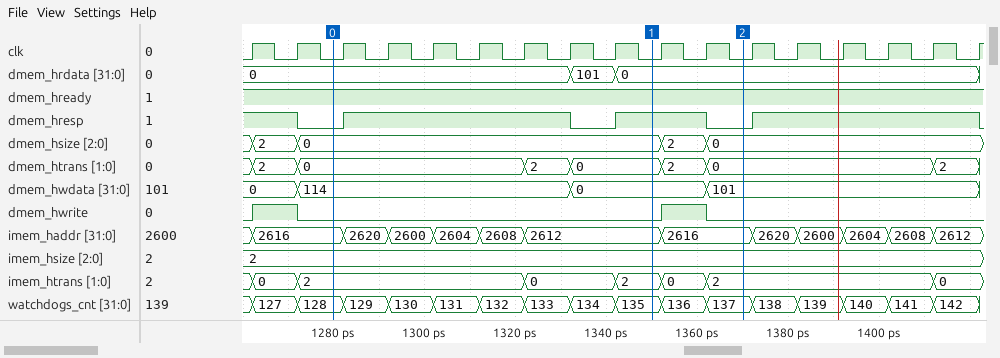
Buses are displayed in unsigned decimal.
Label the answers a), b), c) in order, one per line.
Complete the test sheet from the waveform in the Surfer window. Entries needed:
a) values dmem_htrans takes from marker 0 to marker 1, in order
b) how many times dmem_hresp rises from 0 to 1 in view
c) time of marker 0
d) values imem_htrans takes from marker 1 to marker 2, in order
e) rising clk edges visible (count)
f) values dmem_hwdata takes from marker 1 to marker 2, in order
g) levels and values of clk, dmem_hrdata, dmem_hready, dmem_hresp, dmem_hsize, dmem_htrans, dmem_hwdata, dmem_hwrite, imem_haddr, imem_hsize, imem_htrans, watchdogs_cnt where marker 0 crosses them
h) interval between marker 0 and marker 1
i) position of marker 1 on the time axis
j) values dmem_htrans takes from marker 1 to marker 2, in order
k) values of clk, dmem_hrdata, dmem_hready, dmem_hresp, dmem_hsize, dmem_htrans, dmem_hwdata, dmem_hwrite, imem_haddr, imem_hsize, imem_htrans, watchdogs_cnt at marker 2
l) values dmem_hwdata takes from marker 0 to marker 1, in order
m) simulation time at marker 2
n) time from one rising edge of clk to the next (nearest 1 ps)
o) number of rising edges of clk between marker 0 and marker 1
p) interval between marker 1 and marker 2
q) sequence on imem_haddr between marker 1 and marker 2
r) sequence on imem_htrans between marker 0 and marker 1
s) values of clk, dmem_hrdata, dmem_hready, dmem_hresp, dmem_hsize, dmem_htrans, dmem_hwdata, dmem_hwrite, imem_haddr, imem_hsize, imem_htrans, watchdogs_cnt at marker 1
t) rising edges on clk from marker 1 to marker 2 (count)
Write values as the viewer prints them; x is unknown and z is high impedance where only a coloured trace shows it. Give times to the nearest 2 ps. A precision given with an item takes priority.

a) 0, 2, 0
b) 3
c) 1280 ps
d) 2, 0, 2
e) 17
f) 0, 101
g) clk=0, dmem_hrdata=0, dmem_hready=1, dmem_hresp=0, dmem_hsize=0, dmem_htrans=0, dmem_hwdata=114, dmem_hwrite=0, imem_haddr=2616, imem_hsize=2, imem_htrans=2, watchdogs_cnt=128
h) 70 ps
i) 1350 ps
j) 0, 2, 0
k) clk=0, dmem_hrdata=0, dmem_hready=1, dmem_hresp=0, dmem_hsize=0, dmem_htrans=0, dmem_hwdata=101, dmem_hwrite=0, imem_haddr=2616, imem_hsize=2, imem_htrans=2, watchdogs_cnt=137
l) 114, 0
m) 1370 ps
n) 10 ps
o) 7
p) 20 ps
q) 2612, 2616
r) 2, 0, 2
s) clk=0, dmem_hrdata=0, dmem_hready=1, dmem_hresp=1, dmem_hsize=0, dmem_htrans=0, dmem_hwdata=0, dmem_hwrite=0, imem_haddr=2612, imem_hsize=2, imem_htrans=2, watchdogs_cnt=135
t) 2
